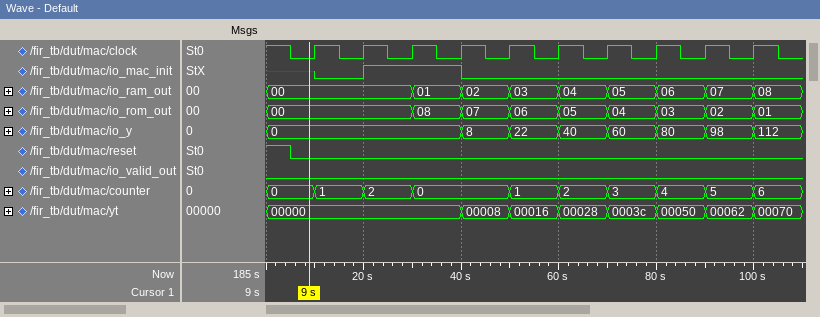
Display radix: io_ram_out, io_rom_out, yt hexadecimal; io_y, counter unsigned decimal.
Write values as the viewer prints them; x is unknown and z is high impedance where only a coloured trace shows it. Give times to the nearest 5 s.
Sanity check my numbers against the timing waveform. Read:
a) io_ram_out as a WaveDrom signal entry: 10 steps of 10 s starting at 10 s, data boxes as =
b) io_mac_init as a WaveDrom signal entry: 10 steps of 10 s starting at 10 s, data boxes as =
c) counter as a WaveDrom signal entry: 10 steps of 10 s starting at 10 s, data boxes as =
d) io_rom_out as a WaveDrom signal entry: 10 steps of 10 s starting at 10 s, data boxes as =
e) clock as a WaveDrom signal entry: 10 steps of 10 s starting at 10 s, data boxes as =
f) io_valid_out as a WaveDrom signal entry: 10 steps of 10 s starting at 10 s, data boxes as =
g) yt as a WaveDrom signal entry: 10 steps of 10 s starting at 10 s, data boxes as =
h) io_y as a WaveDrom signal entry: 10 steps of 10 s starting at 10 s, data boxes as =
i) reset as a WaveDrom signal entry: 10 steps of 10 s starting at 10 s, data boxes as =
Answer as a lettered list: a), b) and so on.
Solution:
a) {name: 'io_ram_out', wave: '=.========', data: '00 01 02 03 04 05 06 07 08'}
b) {name: 'io_mac_init', wave: '01.0......'}
c) {name: 'counter', wave: '===.======', data: '1 2 0 1 2 3 4 5 6'}
d) {name: 'io_rom_out', wave: '=.========', data: '00 08 07 06 05 04 03 02 01'}
e) {name: 'clock', wave: 'p.........'}
f) {name: 'io_valid_out', wave: '0.........'}
g) {name: 'yt', wave: '=..=======', data: '00000 00008 00016 00028 0003c 00050 00062 00070'}
h) {name: 'io_y', wave: '=..=======', data: '0 8 22 40 60 80 98 112'}
i) {name: 'reset', wave: '0.........'}
